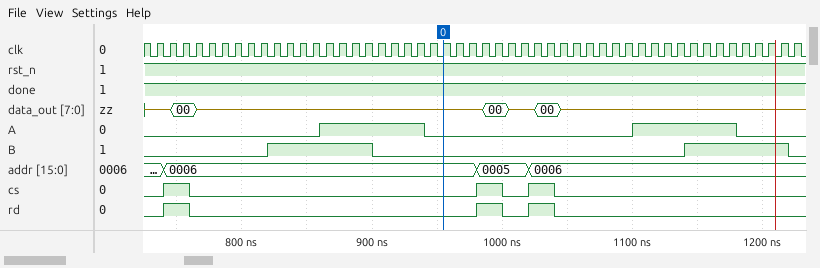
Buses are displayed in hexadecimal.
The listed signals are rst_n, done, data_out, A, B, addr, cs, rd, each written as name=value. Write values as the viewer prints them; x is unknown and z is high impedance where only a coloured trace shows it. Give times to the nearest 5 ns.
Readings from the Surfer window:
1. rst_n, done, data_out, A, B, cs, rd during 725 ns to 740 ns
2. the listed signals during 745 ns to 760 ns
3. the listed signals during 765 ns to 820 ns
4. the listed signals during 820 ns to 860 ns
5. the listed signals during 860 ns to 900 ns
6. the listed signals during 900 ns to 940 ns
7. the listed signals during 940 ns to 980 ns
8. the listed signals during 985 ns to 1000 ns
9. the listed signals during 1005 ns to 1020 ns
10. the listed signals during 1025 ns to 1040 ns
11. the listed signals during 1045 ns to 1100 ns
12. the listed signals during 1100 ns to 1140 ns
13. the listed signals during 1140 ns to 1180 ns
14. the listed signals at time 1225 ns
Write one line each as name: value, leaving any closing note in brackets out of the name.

rst_n, done, data_out, A, B, cs, rd during 725 ns to 740 ns: rst_n=1, done=1, data_out=z, A=0, B=0, cs=0, rd=0
the listed signals during 745 ns to 760 ns: rst_n=1, done=1, data_out=00, A=0, B=0, addr=0006, cs=1, rd=1
the listed signals during 765 ns to 820 ns: rst_n=1, done=1, data_out=z, A=0, B=0, addr=0006, cs=0, rd=0
the listed signals during 820 ns to 860 ns: rst_n=1, done=1, data_out=z, A=0, B=1, addr=0006, cs=0, rd=0
the listed signals during 860 ns to 900 ns: rst_n=1, done=1, data_out=z, A=1, B=1, addr=0006, cs=0, rd=0
the listed signals during 900 ns to 940 ns: rst_n=1, done=1, data_out=z, A=1, B=0, addr=0006, cs=0, rd=0
the listed signals during 940 ns to 980 ns: rst_n=1, done=1, data_out=z, A=0, B=0, addr=0006, cs=0, rd=0
the listed signals during 985 ns to 1000 ns: rst_n=1, done=1, data_out=00, A=0, B=0, addr=0005, cs=1, rd=1
the listed signals during 1005 ns to 1020 ns: rst_n=1, done=1, data_out=z, A=0, B=0, addr=0005, cs=0, rd=0
the listed signals during 1025 ns to 1040 ns: rst_n=1, done=1, data_out=00, A=0, B=0, addr=0006, cs=1, rd=1
the listed signals during 1045 ns to 1100 ns: rst_n=1, done=1, data_out=z, A=0, B=0, addr=0006, cs=0, rd=0
the listed signals during 1100 ns to 1140 ns: rst_n=1, done=1, data_out=z, A=1, B=0, addr=0006, cs=0, rd=0
the listed signals during 1140 ns to 1180 ns: rst_n=1, done=1, data_out=z, A=1, B=1, addr=0006, cs=0, rd=0
the listed signals at time 1225 ns: rst_n=1, done=1, data_out=z, A=0, B=0, addr=0006, cs=0, rd=0
